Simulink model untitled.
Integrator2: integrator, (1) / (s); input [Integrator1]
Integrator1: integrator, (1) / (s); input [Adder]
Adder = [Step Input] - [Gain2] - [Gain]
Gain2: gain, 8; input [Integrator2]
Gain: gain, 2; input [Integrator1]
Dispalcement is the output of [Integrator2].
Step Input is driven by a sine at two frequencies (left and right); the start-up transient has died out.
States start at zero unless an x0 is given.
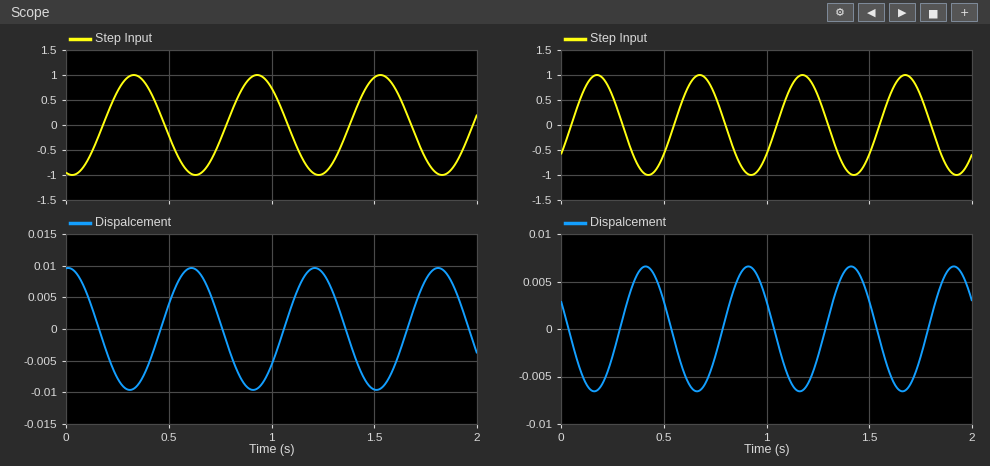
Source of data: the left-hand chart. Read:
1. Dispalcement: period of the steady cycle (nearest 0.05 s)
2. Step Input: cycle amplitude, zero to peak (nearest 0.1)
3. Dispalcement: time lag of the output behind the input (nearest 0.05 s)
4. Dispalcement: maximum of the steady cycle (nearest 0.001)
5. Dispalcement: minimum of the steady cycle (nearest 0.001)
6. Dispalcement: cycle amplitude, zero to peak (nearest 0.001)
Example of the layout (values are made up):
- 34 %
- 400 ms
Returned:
- 0.60 s
- 1.0
- 0.30 s
- 0.010
- -0.010
- 0.010
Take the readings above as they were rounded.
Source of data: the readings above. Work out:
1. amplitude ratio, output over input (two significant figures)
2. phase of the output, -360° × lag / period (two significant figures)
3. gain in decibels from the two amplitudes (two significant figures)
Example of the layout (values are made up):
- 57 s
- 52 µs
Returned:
- 0.010
- -180°
- -40 dB
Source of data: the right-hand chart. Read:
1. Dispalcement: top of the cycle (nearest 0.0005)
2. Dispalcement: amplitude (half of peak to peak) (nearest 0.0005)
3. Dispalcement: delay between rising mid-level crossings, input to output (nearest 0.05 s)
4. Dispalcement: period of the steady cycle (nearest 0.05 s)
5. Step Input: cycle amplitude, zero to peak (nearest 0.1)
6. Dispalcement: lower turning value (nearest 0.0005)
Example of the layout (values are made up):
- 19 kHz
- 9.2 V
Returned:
- 0.0065
- 0.0065
- 0.25 s
- 0.50 s
- 1.0
- -0.0065
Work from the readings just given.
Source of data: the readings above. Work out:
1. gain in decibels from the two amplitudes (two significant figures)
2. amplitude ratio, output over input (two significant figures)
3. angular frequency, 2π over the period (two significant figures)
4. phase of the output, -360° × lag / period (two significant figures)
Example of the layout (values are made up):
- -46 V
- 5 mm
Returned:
- -44 dB
- 0.0065
- 13 rad/s
- -180°
